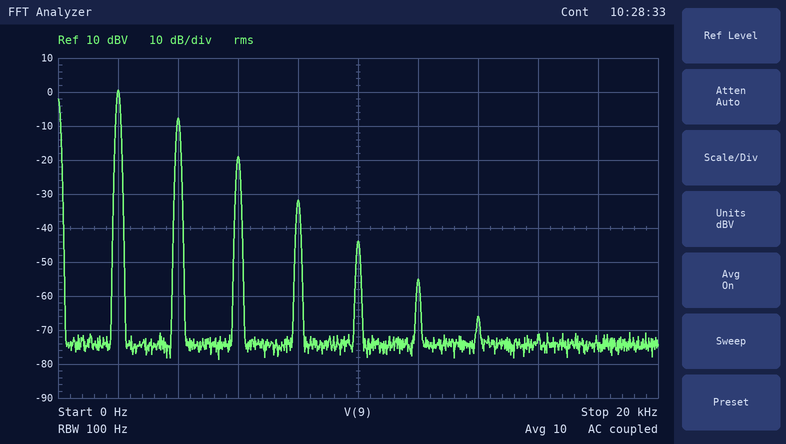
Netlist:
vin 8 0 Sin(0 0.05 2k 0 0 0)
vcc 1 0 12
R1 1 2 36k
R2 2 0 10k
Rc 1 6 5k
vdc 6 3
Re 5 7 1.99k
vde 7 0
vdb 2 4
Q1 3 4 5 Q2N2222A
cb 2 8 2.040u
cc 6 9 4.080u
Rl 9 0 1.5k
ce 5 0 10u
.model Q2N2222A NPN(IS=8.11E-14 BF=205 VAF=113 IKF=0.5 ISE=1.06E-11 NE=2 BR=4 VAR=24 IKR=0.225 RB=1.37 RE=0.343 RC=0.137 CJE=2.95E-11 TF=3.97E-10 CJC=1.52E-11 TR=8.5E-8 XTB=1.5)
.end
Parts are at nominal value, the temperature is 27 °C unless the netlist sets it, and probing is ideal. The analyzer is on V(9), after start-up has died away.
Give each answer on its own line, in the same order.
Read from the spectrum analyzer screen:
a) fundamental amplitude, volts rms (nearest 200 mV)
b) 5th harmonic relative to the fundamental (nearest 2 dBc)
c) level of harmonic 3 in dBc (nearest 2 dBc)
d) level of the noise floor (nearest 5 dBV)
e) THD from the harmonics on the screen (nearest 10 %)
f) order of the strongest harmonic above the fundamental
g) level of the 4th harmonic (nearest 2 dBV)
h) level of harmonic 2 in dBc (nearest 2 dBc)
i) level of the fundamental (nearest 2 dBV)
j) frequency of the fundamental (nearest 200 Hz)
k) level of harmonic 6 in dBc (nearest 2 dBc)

1.0 V
-44 dBc
-20 dBc
-75 dBV
40 %
2
-32 dBV
-8 dBc
0 dBV
2.0 kHz
-56 dBc
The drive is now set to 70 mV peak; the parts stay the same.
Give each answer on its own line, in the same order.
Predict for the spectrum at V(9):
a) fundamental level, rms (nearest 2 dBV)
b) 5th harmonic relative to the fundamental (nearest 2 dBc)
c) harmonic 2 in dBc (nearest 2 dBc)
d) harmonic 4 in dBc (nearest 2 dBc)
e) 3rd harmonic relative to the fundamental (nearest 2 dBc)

2 dBV
-36 dBc
-6 dBc
-26 dBc
-14 dBc
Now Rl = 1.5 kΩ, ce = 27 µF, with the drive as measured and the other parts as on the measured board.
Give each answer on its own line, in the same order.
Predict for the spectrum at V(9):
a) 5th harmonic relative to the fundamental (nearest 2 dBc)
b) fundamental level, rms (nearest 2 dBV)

-48 dBc
0 dBV
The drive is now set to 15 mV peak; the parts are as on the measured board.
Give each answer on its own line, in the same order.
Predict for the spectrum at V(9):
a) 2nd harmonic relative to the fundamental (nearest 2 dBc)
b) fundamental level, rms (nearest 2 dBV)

-18 dBc
-8 dBV
